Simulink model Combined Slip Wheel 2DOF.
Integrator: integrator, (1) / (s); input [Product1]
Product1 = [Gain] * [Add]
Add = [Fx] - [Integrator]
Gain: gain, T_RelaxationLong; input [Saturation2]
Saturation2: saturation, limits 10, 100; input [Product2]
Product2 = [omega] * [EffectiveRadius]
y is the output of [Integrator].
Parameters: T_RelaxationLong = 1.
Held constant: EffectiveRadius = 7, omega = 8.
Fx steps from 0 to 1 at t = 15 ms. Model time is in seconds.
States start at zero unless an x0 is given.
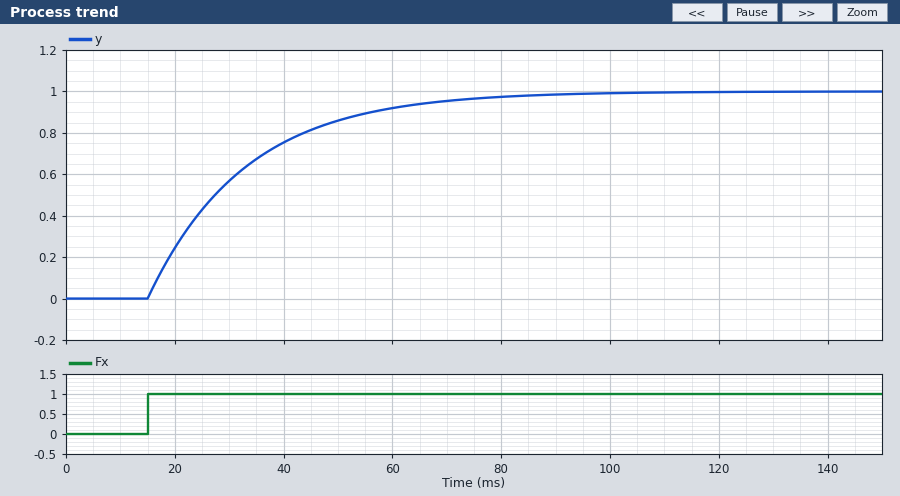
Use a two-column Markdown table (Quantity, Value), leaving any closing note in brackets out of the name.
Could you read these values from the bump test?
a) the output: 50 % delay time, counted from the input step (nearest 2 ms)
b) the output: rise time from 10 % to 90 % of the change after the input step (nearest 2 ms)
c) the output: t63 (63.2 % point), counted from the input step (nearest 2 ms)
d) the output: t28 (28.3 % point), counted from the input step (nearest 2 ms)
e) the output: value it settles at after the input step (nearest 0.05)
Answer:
| Quantity | Value |
|---|---|
| the output: 50 % delay time, counted from the input step | 12 ms |
| the output: rise time from 10 % to 90 % of the change after the input step | 40 ms |
| the output: t63 (63.2 % point), counted from the input step | 18 ms |
| the output: t28 (28.3 % point), counted from the input step | 6 ms |
| the output: value it settles at after the input step | 1.00 |
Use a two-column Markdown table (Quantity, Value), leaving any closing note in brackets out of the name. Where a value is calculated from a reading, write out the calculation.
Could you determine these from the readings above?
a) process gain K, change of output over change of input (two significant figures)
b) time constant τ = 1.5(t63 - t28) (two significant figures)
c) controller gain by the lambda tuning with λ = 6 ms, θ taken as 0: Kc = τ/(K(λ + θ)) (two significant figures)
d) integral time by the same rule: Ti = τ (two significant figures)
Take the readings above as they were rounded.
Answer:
| Quantity | Value |
|---|---|
| process gain K, change of output over change of input | (1 - 0) / 1 = 1.0 |
| time constant τ = 1.5(t63 - t28) | 1.5 × (18 - 6) = 18 ms |
| controller gain by the lambda tuning with λ = 6 ms, θ taken as 0: Kc = τ/(K(λ + θ)) | 18 / (1 × (6 + 0)) = 3.0 |
| integral time by the same rule: Ti = τ | 18 ms |
